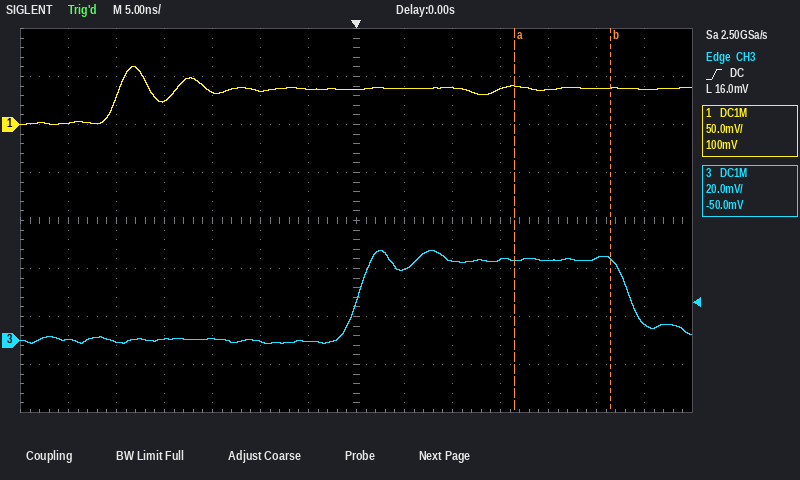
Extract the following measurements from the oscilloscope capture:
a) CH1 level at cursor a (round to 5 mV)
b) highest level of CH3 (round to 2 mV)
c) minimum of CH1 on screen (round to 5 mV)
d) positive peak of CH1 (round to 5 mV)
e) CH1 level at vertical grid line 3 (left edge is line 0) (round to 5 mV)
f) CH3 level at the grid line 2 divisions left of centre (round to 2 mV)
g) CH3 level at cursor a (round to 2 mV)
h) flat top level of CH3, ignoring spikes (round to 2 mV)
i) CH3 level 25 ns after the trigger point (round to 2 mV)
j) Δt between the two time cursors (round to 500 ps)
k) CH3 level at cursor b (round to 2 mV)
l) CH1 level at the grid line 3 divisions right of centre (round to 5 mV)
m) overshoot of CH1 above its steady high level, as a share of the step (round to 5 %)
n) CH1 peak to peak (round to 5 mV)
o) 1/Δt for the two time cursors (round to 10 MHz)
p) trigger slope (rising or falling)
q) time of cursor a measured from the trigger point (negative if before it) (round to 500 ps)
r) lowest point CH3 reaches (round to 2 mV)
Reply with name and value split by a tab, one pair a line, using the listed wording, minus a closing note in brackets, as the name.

CH1 level at cursor a	40 mV
highest level of CH3	38 mV
minimum of CH1 on screen	0 mV
positive peak of CH1	60 mV
CH1 level at vertical grid line 3 (left edge is line 0)	25 mV
CH3 level at the grid line 2 divisions left of centre	0 mV
CH3 level at cursor a	34 mV
flat top level of CH3, ignoring spikes	34 mV
CH3 level 25 ns after the trigger point	34 mV
Δt between the two time cursors	10.0 ns
CH3 level at cursor b	34 mV
CH1 level at the grid line 3 divisions right of centre	35 mV
overshoot of CH1 above its steady high level, as a share of the step	65 %
CH1 peak to peak	60 mV
1/Δt for the two time cursors	100 MHz
trigger slope	rising
time of cursor a measured from the trigger point (negative if before it)	+16.5 ns
lowest point CH3 reaches	-2 mV
